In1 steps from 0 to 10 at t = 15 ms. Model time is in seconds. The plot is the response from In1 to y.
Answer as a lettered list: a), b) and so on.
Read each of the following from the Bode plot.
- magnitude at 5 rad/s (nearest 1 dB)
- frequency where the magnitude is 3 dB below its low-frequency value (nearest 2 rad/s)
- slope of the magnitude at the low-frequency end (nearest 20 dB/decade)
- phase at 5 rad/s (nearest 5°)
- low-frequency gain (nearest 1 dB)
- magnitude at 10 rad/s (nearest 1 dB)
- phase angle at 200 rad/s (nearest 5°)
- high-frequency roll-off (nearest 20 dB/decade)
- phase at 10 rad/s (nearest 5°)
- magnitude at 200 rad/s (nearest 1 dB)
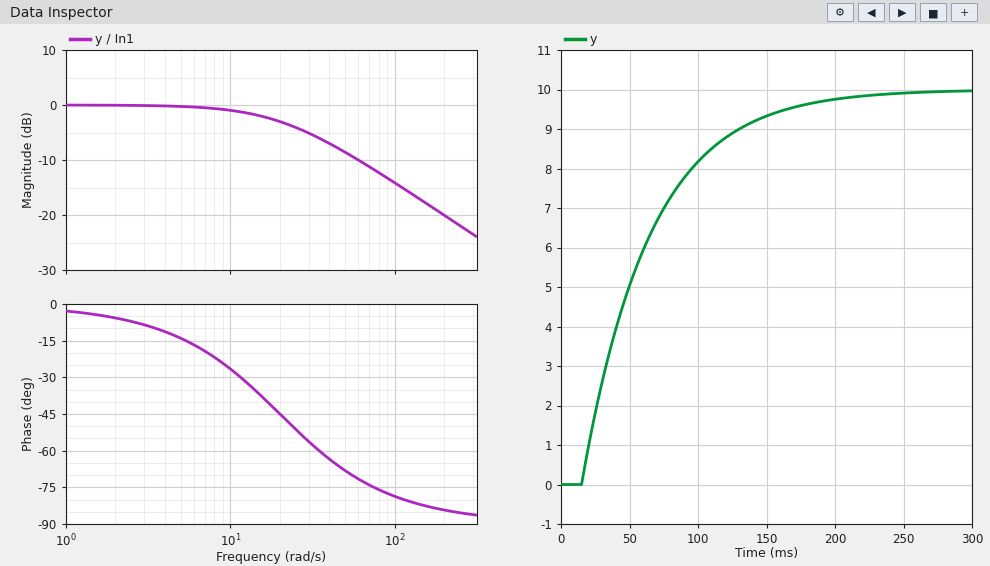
a) 0 dB
b) 20 rad/s
c) 0 dB/decade
d) -15°
e) 0 dB
f) -1 dB
g) -85°
h) -20 dB/decade
i) -25°
j) -20 dB
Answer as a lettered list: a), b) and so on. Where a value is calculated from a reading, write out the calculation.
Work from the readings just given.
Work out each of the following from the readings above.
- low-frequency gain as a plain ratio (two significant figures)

a) 10^(0 / 20) = 1.0
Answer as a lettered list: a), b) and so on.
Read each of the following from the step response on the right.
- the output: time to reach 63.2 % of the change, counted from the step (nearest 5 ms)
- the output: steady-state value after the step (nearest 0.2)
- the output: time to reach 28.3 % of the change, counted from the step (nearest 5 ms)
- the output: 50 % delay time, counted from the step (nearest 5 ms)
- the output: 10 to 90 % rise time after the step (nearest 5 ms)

a) 50 ms
b) 10.0
c) 15 ms
d) 35 ms
e) 110 ms
